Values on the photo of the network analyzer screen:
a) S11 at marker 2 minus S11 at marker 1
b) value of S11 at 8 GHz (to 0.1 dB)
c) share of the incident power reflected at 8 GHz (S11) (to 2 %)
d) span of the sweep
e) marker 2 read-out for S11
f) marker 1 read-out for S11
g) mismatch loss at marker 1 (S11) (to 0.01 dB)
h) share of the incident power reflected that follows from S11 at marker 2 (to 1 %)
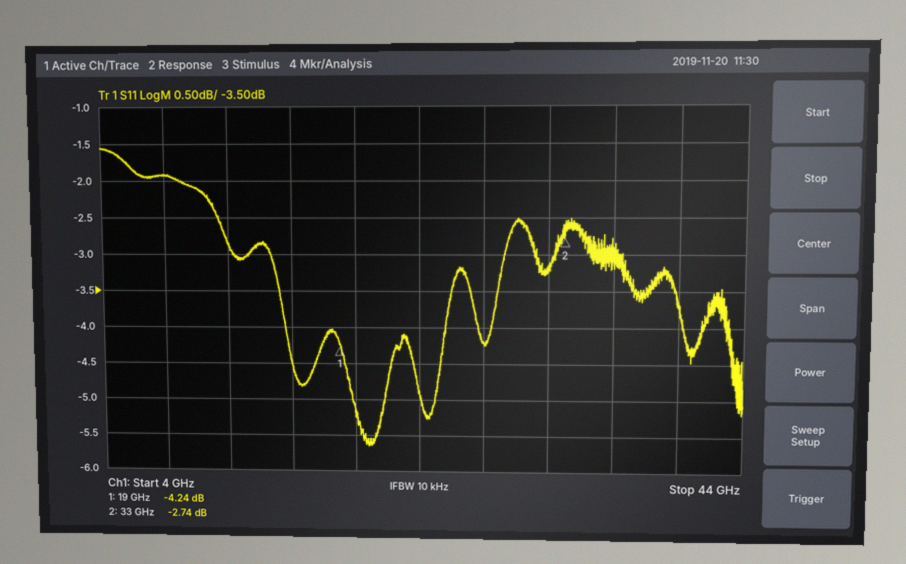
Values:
1.50 dB
-1.9 dB
64 %
40 GHz
-2.74 dB
-4.24 dB
2.05 dB
53 %
